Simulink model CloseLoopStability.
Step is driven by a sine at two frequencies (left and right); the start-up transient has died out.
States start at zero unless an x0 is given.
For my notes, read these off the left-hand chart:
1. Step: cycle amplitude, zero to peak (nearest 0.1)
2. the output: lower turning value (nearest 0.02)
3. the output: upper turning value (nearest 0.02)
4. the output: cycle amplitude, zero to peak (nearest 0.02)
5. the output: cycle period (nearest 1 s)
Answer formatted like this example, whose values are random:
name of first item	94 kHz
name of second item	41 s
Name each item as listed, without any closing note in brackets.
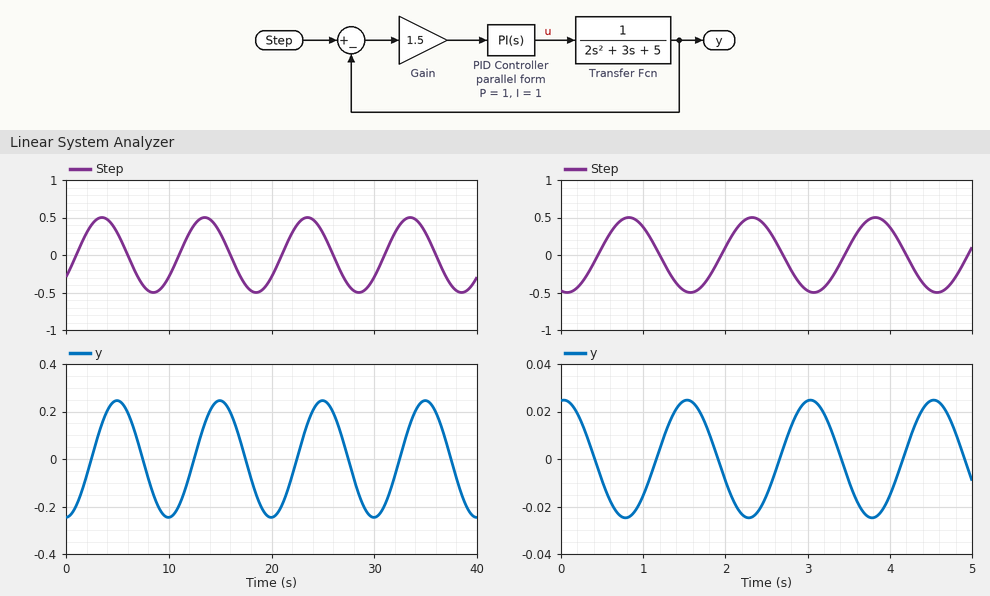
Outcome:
Step: cycle amplitude, zero to peak	0.5
the output: lower turning value	-0.24
the output: upper turning value	0.24
the output: cycle amplitude, zero to peak	0.24
the output: cycle period	10 s
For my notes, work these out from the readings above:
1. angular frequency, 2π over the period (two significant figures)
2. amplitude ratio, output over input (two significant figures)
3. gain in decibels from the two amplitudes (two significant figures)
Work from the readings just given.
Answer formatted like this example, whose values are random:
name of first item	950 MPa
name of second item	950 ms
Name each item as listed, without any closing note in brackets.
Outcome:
angular frequency, 2π over the period	0.63 rad/s
amplitude ratio, output over input	0.48
gain in decibels from the two amplitudes	-6.4 dB
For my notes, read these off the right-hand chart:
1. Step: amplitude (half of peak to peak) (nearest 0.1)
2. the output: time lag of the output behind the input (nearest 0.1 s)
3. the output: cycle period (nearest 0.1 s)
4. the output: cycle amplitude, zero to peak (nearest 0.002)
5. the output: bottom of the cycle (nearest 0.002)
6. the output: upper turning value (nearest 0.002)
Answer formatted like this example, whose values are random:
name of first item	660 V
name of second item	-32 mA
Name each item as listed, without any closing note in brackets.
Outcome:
Step: amplitude (half of peak to peak)	0.5
the output: time lag of the output behind the input	0.7 s
the output: cycle period	1.5 s
the output: cycle amplitude, zero to peak	0.024
the output: bottom of the cycle	-0.024
the output: upper turning value	0.024
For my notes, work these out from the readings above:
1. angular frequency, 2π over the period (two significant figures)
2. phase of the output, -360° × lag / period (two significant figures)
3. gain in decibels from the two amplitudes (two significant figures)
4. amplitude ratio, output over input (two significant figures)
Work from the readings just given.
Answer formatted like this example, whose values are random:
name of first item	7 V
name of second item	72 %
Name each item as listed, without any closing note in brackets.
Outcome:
angular frequency, 2π over the period	4.2 rad/s
phase of the output, -360° × lag / period	-170°
gain in decibels from the two amplitudes	-26 dB
amplitude ratio, output over input	0.048
